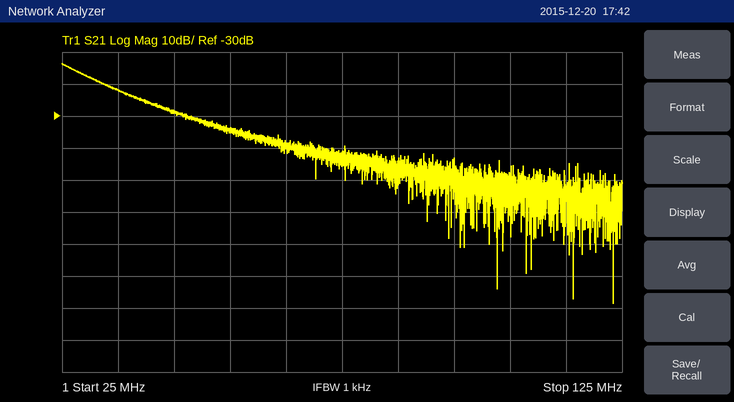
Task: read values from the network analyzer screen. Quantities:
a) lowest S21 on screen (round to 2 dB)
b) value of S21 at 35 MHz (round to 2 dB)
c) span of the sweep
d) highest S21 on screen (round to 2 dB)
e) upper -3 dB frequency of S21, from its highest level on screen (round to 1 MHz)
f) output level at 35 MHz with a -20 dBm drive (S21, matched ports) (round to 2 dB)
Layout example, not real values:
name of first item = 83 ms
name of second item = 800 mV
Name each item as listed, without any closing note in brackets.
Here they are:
lowest S21 on screen = -88 dB
value of S21 at 35 MHz = -22 dB
span of the sweep = 100 MHz
highest S21 on screen = -14 dB
upper -3 dB frequency of S21, from its highest level on screen = 28 MHz
output level at 35 MHz with a -20 dBm drive (S21, matched ports) = -42 dBm
